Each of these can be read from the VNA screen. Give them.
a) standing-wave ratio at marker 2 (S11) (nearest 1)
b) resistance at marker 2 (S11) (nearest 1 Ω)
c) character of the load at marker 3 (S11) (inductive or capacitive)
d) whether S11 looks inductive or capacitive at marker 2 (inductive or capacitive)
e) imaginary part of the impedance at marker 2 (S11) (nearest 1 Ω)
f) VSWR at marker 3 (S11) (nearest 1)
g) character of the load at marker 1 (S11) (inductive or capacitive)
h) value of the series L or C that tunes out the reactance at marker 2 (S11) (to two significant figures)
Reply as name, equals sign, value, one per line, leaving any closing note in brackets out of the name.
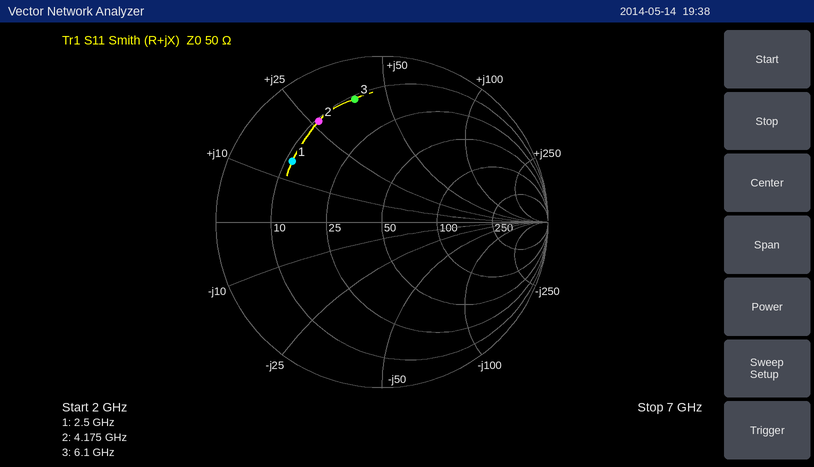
standing-wave ratio at marker 2 (S11) = 6
resistance at marker 2 (S11) = 11 Ω
character of the load at marker 3 (S11) = inductive
whether S11 looks inductive or capacitive at marker 2 = inductive
imaginary part of the impedance at marker 2 (S11) = +27 Ω
VSWR at marker 3 (S11) = 7
character of the load at marker 1 (S11) = inductive
value of the series L or C that tunes out the reactance at marker 2 (S11) = 1.4 pF
